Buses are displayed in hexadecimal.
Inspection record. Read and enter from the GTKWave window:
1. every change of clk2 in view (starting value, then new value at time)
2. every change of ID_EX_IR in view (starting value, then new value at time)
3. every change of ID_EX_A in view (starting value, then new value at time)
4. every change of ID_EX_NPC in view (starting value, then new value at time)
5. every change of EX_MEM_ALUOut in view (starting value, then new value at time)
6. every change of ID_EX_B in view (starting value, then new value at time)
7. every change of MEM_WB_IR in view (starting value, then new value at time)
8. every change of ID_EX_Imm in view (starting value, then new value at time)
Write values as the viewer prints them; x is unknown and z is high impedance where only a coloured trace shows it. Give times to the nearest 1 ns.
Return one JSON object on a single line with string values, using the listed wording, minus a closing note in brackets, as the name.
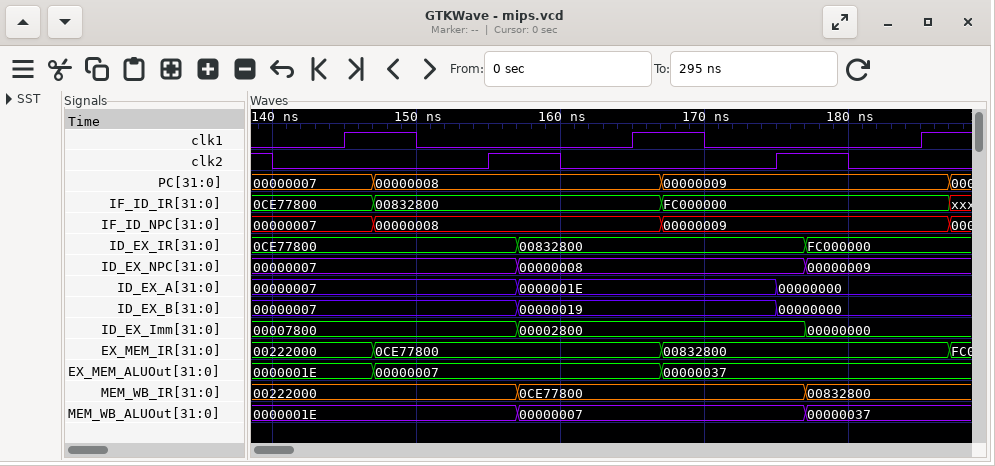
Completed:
{"every change of clk2 in view": "1, 0 at 140 ns, 1 at 155 ns, 0 at 160 ns, 1 at 175 ns, 0 at 180 ns", "every change of ID_EX_IR in view": "0CE77800, 00832800 at 157 ns, FC000000 at 177 ns", "every change of ID_EX_A in view": "00000007, 0000001E at 157 ns, 00000000 at 175 ns", "every change of ID_EX_NPC in view": "00000007, 00000008 at 157 ns, 00000009 at 177 ns", "every change of EX_MEM_ALUOut in view": "0000001E, 00000007 at 147 ns, 00000037 at 167 ns", "every change of ID_EX_B in view": "00000007, 00000019 at 157 ns, 00000000 at 175 ns", "every change of MEM_WB_IR in view": "00222000, 0CE77800 at 157 ns, 00832800 at 177 ns", "every change of ID_EX_Imm in view": "00007800, 00002800 at 157 ns, 00000000 at 177 ns"}
